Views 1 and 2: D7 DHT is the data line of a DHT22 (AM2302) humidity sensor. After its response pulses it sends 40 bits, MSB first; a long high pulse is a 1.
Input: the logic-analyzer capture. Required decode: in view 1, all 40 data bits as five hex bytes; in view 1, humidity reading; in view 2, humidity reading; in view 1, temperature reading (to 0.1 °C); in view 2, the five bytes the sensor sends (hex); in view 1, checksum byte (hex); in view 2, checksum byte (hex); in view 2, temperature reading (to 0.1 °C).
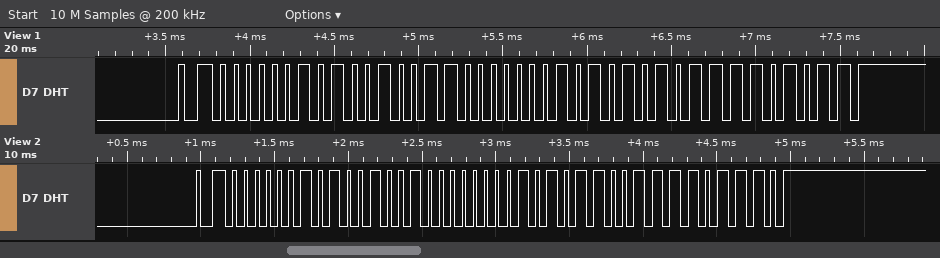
02 93 01 55 EB
65.9 %
65.8 %
34.1 °C
02 92 01 59 EE
0xEB
0xEE
34.5 °C
